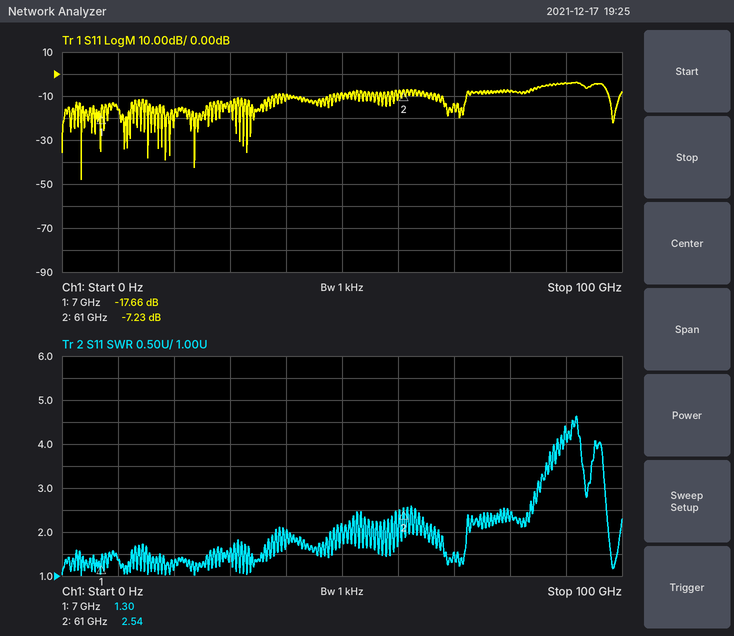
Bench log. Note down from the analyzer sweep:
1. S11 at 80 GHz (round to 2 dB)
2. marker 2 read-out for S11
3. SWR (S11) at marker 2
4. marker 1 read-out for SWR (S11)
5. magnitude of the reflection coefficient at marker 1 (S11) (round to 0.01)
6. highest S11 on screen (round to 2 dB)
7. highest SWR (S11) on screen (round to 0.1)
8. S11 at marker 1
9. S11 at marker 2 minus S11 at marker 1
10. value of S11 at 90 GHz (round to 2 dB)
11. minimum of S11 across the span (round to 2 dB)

-8 dB
-7.23 dB
2.54
1.30
0.13
-4 dB
4.6
-17.66 dB
10.43 dB
-4 dB
-48 dB
